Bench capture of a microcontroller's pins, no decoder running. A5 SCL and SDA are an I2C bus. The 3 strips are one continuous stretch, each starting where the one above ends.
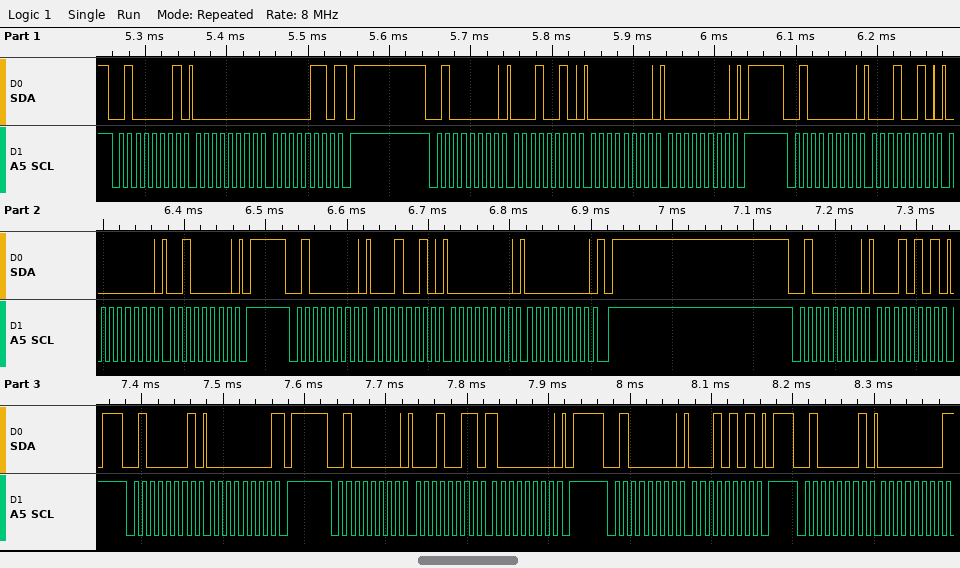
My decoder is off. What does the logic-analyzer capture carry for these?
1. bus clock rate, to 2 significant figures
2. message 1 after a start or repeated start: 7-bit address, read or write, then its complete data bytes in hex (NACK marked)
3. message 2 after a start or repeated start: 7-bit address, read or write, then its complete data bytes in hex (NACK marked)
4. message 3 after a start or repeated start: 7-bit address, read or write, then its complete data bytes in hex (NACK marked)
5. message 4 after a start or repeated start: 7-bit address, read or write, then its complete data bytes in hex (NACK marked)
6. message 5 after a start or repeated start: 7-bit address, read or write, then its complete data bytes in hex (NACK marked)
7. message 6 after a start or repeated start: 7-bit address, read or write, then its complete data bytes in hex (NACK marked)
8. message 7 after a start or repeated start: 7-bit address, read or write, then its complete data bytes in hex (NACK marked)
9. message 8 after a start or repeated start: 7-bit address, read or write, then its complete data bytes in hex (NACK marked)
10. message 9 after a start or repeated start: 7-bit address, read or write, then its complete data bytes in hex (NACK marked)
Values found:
100 kHz
0x20 read: 00 06 NACK
0x20 write: 12 00 00
0x20 write: 12 00 20
0x20 write: 12 00 00
0x20 write: 15
0x20 read: 00 NACK
0x20 write: 13 80
0x20 write: 15
0x20 read: 00 NACK
